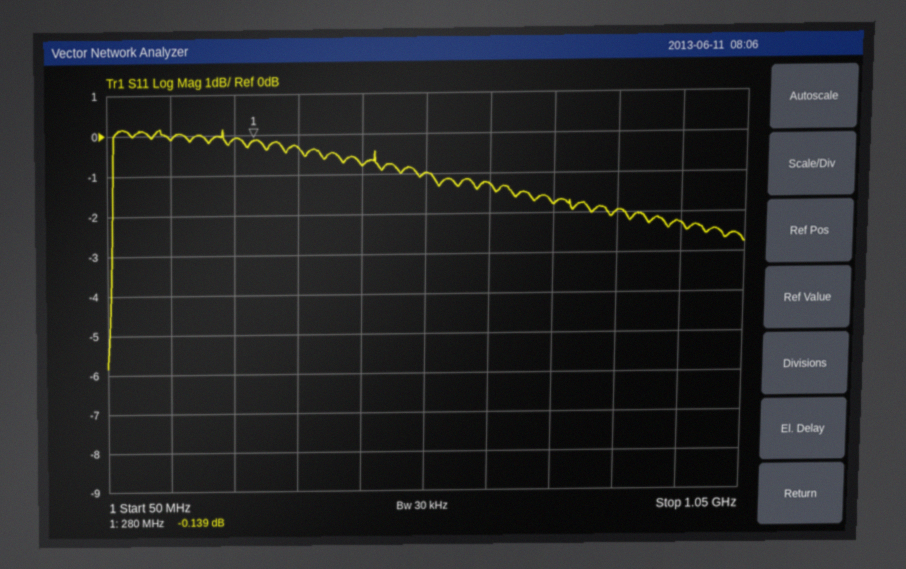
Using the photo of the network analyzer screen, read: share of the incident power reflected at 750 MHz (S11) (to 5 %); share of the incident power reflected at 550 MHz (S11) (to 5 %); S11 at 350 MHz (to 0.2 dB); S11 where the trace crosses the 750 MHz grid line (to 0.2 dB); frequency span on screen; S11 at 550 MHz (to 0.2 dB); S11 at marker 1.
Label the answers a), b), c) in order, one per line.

a) 65 %
b) 80 %
c) -0.4 dB
d) -1.8 dB
e) 1 GHz
f) -1.0 dB
g) -0.139 dB
